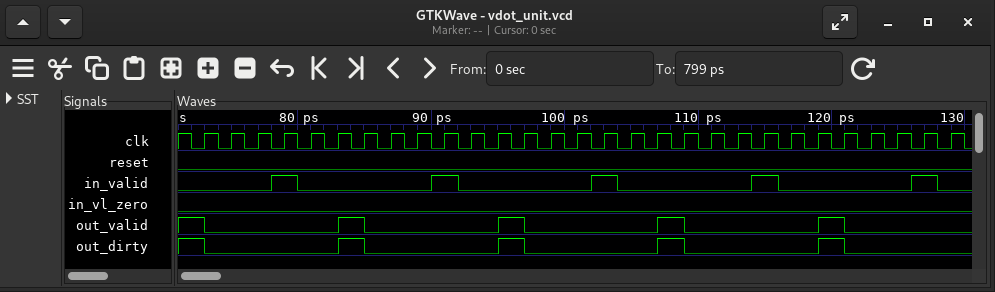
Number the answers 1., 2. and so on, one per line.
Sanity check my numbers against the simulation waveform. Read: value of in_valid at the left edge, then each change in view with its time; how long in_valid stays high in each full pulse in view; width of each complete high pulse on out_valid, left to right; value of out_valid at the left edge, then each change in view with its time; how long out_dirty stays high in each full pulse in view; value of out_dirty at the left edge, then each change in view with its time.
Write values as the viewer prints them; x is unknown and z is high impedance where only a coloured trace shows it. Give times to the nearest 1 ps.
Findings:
1. 0, 1 at 78 ps, 0 at 80 ps, 1 at 90 ps, 0 at 92 ps, 1 at 102 ps, 0 at 104 ps, 1 at 114 ps, 0 at 116 ps, 1 at 126 ps, 0 at 128 ps
2. 2 ps, 2 ps, 2 ps, 2 ps, 2 ps
3. 2 ps, 2 ps, 2 ps, 2 ps
4. 1, 0 at 73 ps, 1 at 83 ps, 0 at 85 ps, 1 at 95 ps, 0 at 97 ps, 1 at 107 ps, 0 at 109 ps, 1 at 119 ps, 0 at 121 ps
5. 2 ps, 2 ps, 2 ps, 2 ps
6. 1, 0 at 73 ps, 1 at 83 ps, 0 at 85 ps, 1 at 95 ps, 0 at 97 ps, 1 at 107 ps, 0 at 109 ps, 1 at 119 ps, 0 at 121 ps
